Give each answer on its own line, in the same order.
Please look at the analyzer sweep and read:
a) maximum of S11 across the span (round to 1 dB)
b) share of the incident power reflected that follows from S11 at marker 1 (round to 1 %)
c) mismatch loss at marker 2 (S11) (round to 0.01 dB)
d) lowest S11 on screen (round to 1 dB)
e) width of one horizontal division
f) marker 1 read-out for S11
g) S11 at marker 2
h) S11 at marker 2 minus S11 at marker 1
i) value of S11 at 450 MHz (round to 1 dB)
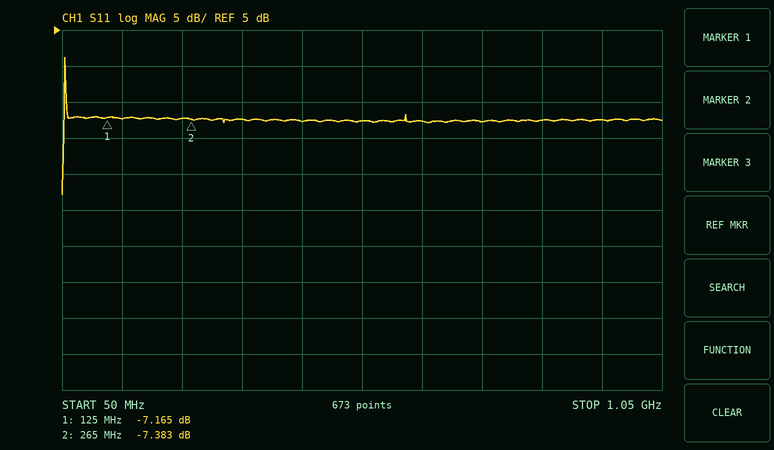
1 dB
19 %
0.88 dB
-18 dB
100 MHz
-7.165 dB
-7.383 dB
-0.218 dB
-8 dB
